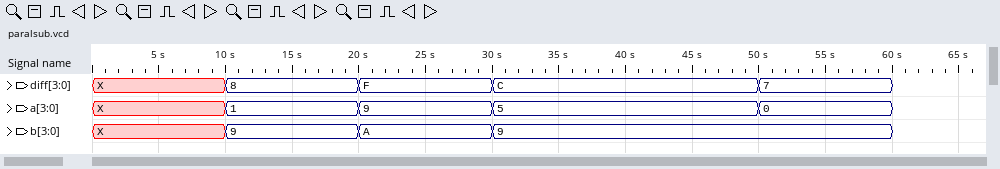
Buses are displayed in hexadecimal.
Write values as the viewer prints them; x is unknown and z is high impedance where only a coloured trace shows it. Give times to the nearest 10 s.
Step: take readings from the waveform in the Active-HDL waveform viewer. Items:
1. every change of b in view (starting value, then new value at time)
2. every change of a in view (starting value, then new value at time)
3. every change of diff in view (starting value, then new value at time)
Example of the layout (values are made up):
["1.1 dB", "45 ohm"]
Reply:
["X, 9 at 10 s, A at 20 s, 9 at 30 s", "X, 1 at 10 s, 9 at 20 s, 5 at 30 s, 0 at 50 s", "X, 8 at 10 s, F at 20 s, C at 30 s, 7 at 50 s"]
